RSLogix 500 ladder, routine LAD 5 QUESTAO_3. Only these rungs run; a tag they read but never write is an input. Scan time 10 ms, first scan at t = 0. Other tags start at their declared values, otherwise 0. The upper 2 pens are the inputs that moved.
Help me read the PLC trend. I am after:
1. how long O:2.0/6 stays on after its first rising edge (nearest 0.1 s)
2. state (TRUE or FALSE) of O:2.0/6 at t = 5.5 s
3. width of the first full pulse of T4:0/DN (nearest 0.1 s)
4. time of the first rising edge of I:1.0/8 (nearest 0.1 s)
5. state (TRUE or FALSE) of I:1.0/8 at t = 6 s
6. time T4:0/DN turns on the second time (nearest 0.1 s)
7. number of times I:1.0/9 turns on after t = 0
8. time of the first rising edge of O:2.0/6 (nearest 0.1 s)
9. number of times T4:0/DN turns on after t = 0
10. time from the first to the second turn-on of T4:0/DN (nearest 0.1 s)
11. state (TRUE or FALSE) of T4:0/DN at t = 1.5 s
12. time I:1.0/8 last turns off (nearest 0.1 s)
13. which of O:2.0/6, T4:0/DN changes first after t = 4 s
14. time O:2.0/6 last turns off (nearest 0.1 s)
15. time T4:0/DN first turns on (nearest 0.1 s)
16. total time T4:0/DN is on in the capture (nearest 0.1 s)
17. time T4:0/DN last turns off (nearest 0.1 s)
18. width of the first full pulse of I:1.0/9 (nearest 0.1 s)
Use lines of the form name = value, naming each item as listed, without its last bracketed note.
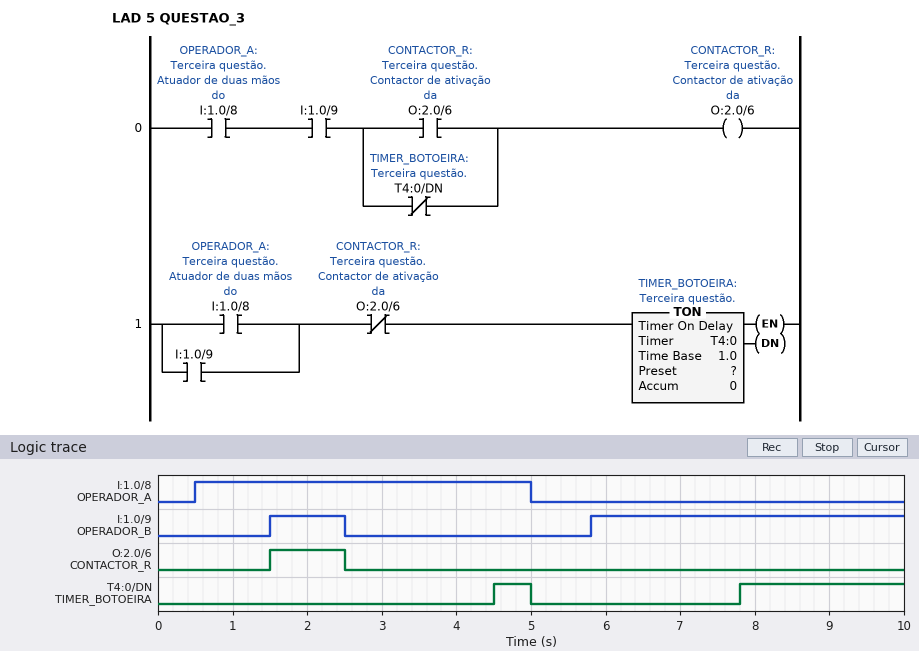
how long O:2.0/6 stays on after its first rising edge = 1.0 s
state (TRUE or FALSE) of O:2.0/6 at t = 5.5 s = FALSE
width of the first full pulse of T4:0/DN = 0.5 s
time of the first rising edge of I:1.0/8 = 0.5 s
state (TRUE or FALSE) of I:1.0/8 at t = 6 s = FALSE
time T4:0/DN turns on the second time = 7.8 s
number of times I:1.0/9 turns on after t = 0 = 2
time of the first rising edge of O:2.0/6 = 1.5 s
number of times T4:0/DN turns on after t = 0 = 2
time from the first to the second turn-on of T4:0/DN = 3.3 s
state (TRUE or FALSE) of T4:0/DN at t = 1.5 s = FALSE
time I:1.0/8 last turns off = 5.0 s
which of O:2.0/6, T4:0/DN changes first after t = 4 s = T4:0/DN
time O:2.0/6 last turns off = 2.5 s
time T4:0/DN first turns on = 4.5 s
total time T4:0/DN is on in the capture = 2.7 s
time T4:0/DN last turns off = 5.0 s
width of the first full pulse of I:1.0/9 = 1.0 s
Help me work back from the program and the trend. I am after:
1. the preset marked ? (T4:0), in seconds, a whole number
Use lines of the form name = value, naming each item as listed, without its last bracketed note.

the preset marked ? (T4:0), in seconds, a whole number = 2 s
